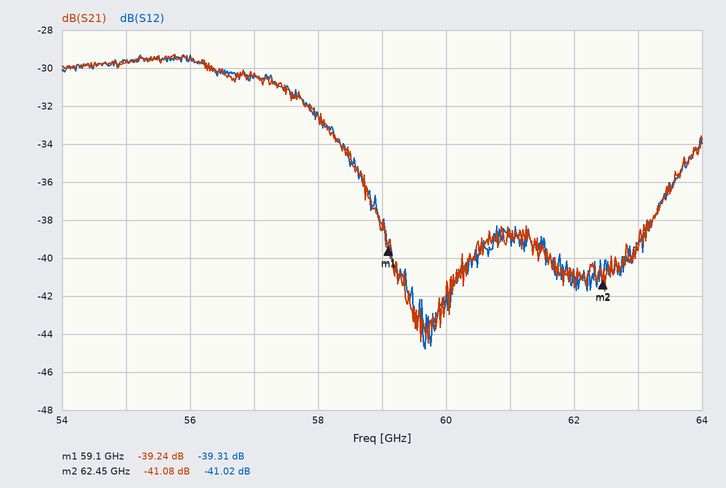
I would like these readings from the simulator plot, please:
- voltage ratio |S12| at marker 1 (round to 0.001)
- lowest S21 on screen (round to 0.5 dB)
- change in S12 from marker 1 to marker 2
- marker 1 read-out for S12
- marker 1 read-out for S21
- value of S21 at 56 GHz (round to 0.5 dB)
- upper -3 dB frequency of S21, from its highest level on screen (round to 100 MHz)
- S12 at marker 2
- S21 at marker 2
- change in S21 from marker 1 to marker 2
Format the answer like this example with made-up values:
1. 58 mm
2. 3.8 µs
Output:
1. 0.011
2. -44.5 dB
3. -1.71 dB
4. -39.31 dB
5. -39.24 dB
6. -29.5 dB
7. 57.9 GHz
8. -41.02 dB
9. -41.08 dB
10. -1.84 dB
